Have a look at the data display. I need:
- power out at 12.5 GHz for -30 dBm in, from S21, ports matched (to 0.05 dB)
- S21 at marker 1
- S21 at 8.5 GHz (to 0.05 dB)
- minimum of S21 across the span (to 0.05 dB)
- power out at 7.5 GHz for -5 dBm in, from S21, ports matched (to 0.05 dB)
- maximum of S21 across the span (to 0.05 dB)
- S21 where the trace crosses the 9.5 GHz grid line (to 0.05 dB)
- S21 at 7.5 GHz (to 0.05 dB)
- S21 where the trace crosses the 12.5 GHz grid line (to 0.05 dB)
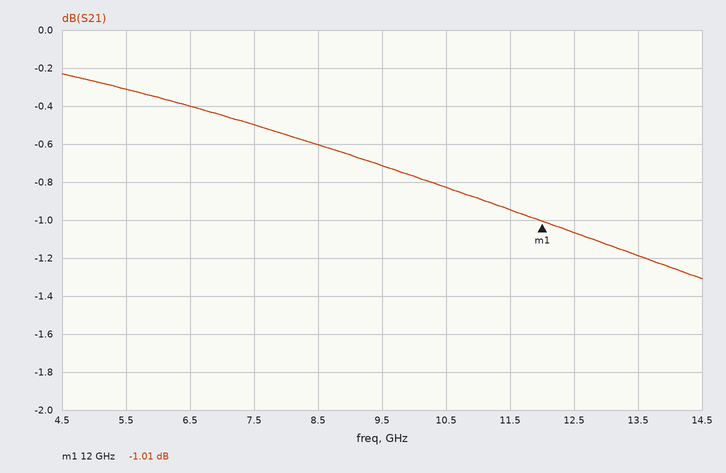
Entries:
-31.05 dBm
-1.01 dB
-0.60 dB
-1.30 dB
-5.50 dBm
-0.25 dB
-0.70 dB
-0.50 dB
-1.05 dB
